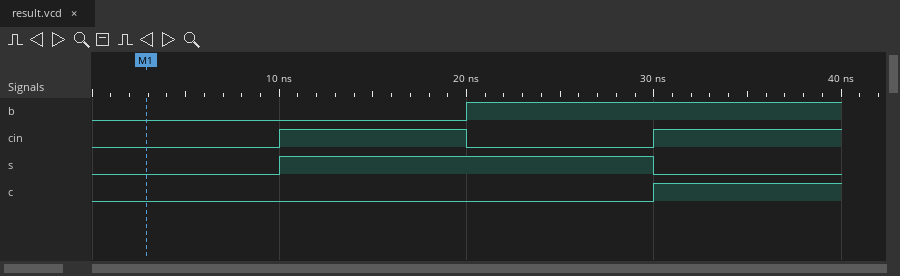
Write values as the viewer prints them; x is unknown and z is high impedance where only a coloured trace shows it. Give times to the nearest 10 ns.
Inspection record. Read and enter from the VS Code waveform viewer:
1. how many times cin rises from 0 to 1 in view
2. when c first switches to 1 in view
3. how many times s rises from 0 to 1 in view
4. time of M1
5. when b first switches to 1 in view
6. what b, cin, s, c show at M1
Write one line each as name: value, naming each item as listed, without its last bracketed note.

how many times cin rises from 0 to 1 in view: 2
when c first switches to 1 in view: 30 ns
how many times s rises from 0 to 1 in view: 1
time of M1: 0 ns
when b first switches to 1 in view: 20 ns
what b, cin, s, c show at M1: b=0, cin=0, s=0, c=0
